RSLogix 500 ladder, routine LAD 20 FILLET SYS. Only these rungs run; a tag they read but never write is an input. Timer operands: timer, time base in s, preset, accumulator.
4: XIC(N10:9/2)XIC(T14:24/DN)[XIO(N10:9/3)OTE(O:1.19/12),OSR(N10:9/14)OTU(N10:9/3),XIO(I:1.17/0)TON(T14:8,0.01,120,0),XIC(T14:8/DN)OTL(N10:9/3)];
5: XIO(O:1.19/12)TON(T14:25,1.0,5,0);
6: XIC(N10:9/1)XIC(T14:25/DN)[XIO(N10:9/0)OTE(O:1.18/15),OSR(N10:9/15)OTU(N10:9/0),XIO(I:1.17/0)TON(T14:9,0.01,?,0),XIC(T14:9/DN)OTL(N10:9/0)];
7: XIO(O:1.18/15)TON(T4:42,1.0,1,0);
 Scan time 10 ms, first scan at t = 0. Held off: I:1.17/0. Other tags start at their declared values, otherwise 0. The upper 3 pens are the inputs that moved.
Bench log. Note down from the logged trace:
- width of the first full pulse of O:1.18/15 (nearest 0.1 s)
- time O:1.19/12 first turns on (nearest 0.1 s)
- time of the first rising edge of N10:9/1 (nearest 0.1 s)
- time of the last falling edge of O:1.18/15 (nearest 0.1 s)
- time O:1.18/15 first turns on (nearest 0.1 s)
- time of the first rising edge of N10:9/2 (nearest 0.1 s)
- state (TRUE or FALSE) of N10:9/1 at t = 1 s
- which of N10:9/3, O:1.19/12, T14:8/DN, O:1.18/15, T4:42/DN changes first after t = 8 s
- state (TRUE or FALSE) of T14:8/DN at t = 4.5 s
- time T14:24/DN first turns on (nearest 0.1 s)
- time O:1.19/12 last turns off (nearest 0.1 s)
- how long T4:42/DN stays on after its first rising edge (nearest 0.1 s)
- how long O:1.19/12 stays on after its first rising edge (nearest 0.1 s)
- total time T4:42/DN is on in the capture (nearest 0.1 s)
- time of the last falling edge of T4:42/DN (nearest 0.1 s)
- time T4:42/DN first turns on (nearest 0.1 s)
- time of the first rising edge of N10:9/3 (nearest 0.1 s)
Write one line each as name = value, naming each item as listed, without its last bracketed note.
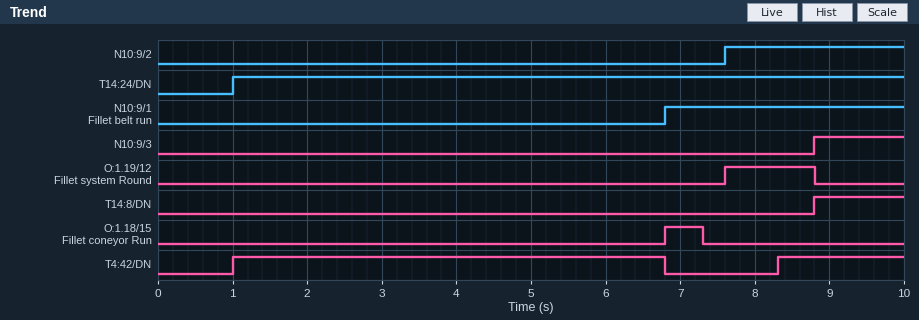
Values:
width of the first full pulse of O:1.18/15 = 0.5 s
time O:1.19/12 first turns on = 7.6 s
time of the first rising edge of N10:9/1 = 6.8 s
time of the last falling edge of O:1.18/15 = 7.3 s
time O:1.18/15 first turns on = 6.8 s
time of the first rising edge of N10:9/2 = 7.6 s
state (TRUE or FALSE) of N10:9/1 at t = 1 s = FALSE
which of N10:9/3, O:1.19/12, T14:8/DN, O:1.18/15, T4:42/DN changes first after t = 8 s = T4:42/DN
state (TRUE or FALSE) of T14:8/DN at t = 4.5 s = FALSE
time T14:24/DN first turns on = 1.0 s
time O:1.19/12 last turns off = 8.8 s
how long T4:42/DN stays on after its first rising edge = 5.8 s
how long O:1.19/12 stays on after its first rising edge = 1.2 s
total time T4:42/DN is on in the capture = 7.5 s
time of the last falling edge of T4:42/DN = 6.8 s
time T4:42/DN first turns on = 1.0 s
time of the first rising edge of N10:9/3 = 8.8 s
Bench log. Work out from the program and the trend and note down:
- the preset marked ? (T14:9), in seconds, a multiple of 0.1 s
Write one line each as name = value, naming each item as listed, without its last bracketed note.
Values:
the preset marked ? (T14:9), in seconds, a multiple of 0.1 s = 0.5 s
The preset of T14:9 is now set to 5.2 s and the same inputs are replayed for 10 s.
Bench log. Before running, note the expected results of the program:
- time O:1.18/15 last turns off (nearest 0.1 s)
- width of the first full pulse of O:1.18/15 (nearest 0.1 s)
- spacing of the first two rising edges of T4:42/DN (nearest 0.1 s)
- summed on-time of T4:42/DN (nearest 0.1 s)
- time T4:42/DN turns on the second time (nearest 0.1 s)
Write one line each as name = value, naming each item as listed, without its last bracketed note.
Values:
time O:1.18/15 last turns off = 7.6 s
width of the first full pulse of O:1.18/15 = 0.8 s
spacing of the first two rising edges of T4:42/DN = 7.6 s
summed on-time of T4:42/DN = 7.2 s
time T4:42/DN turns on the second time = 8.6 s
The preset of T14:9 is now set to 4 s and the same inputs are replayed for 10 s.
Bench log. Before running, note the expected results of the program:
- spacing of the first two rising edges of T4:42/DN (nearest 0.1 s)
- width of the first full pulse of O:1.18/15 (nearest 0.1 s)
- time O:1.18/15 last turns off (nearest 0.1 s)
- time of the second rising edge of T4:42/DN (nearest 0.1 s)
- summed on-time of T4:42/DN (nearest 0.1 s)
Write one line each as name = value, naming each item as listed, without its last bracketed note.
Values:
spacing of the first two rising edges of T4:42/DN = 7.6 s
width of the first full pulse of O:1.18/15 = 0.8 s
time O:1.18/15 last turns off = 7.6 s
time of the second rising edge of T4:42/DN = 8.6 s
summed on-time of T4:42/DN = 7.2 s
